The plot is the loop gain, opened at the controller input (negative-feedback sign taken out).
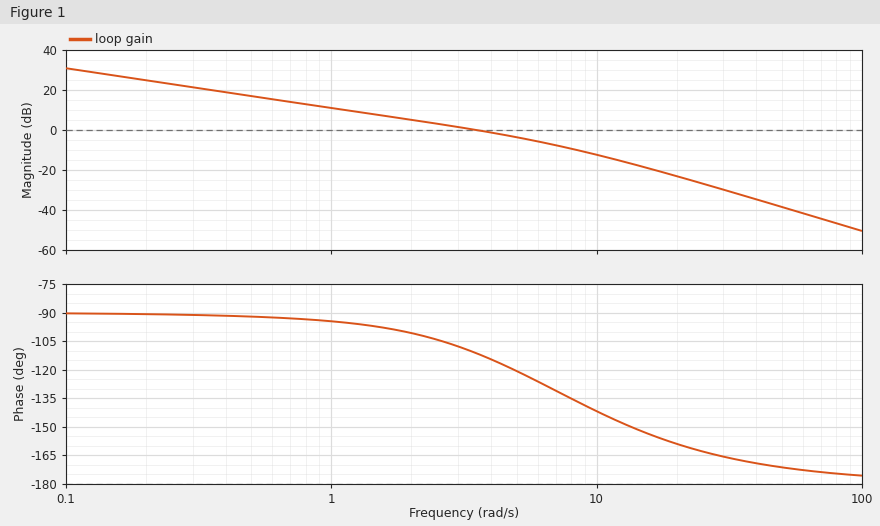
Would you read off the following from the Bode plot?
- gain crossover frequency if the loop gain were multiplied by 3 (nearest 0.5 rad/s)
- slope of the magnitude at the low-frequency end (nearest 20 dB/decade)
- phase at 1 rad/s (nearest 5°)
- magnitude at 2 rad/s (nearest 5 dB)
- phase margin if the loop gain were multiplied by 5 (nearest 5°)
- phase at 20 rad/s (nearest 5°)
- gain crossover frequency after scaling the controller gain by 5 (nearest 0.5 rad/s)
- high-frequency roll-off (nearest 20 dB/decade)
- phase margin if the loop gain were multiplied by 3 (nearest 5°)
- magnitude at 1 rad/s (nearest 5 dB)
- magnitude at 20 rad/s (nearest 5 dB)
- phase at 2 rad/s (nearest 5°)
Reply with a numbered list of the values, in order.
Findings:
1. 8.0 rad/s
2. -20 dB/decade
3. -95°
4. 5 dB
5. 35°
6. -160°
7. 11.0 rad/s
8. -40 dB/decade
9. 45°
10. 10 dB
11. -25 dB
12. -100°
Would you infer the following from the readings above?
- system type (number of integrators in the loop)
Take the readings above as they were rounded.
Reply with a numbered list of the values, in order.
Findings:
1. 1
